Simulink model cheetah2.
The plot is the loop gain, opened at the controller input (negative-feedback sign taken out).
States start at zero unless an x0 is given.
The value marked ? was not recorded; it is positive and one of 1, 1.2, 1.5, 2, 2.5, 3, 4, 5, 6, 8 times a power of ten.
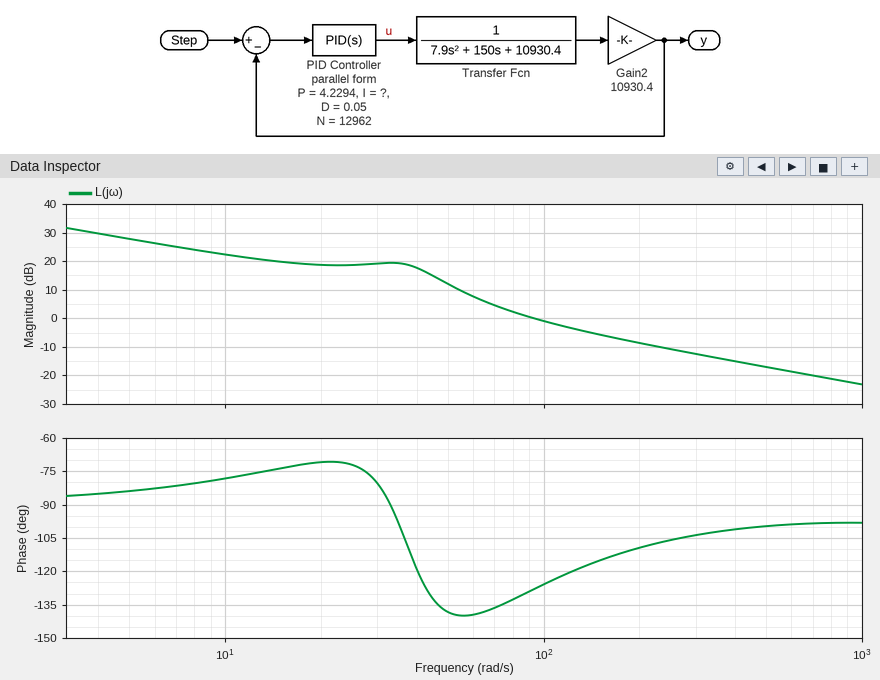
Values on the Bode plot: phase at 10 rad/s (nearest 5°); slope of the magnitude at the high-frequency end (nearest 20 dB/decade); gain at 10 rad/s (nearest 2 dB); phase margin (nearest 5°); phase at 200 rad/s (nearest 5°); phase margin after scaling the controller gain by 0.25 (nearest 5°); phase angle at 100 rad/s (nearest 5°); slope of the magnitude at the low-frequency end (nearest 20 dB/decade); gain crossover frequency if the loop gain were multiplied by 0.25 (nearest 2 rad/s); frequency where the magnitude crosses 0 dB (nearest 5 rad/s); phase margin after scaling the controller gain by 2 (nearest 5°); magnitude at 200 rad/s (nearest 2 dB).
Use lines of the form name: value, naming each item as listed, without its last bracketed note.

phase at 10 rad/s: -80°
slope of the magnitude at the high-frequency end: -20 dB/decade
gain at 10 rad/s: 22 dB
phase margin: 50°
phase at 200 rad/s: -110°
phase margin after scaling the controller gain by 0.25: 40°
phase angle at 100 rad/s: -125°
slope of the magnitude at the low-frequency end: -20 dB/decade
gain crossover frequency if the loop gain were multiplied by 0.25: 50 rad/s
frequency where the magnitude crosses 0 dB: 95 rad/s
phase margin after scaling the controller gain by 2: 65°
magnitude at 200 rad/s: -8 dB
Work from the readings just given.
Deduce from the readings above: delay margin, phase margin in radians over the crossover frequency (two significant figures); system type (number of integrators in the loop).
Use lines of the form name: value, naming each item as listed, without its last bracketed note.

delay margin, phase margin in radians over the crossover frequency: 0.0092 s
system type: 1
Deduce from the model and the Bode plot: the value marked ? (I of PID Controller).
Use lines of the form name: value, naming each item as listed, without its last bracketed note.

the value marked ?: 120
